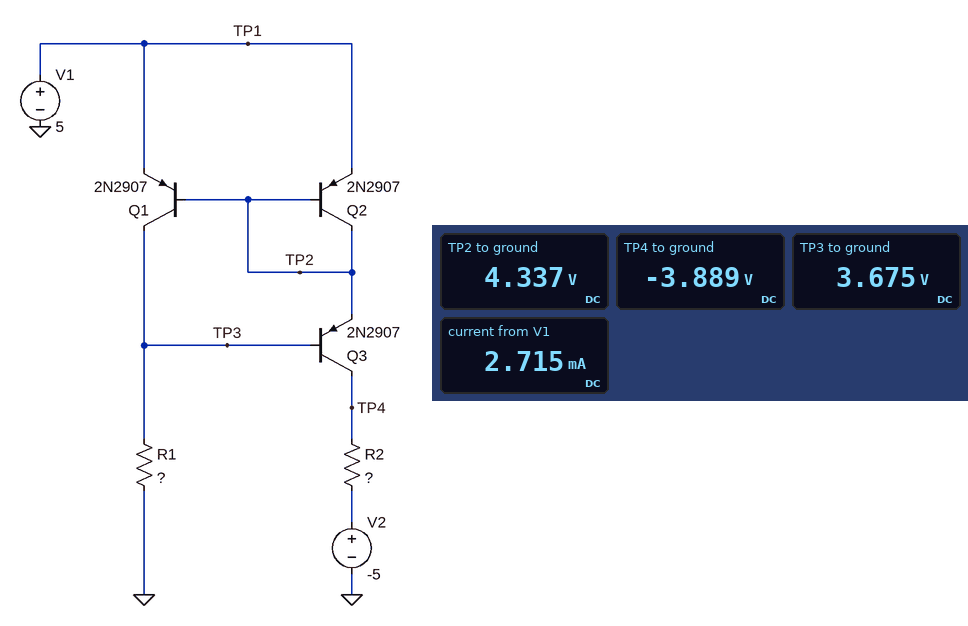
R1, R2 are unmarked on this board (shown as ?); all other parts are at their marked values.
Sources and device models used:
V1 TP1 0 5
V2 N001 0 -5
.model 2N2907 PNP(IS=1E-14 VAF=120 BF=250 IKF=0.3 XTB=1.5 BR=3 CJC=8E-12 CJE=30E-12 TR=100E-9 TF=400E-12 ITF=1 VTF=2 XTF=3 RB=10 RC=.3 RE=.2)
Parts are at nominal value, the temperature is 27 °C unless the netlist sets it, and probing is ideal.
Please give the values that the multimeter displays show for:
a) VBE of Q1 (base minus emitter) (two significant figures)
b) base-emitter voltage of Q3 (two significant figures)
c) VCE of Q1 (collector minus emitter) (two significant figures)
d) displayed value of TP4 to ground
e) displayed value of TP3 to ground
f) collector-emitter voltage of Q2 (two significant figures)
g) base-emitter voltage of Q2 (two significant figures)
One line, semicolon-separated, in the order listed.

-660 mV; -660 mV; -1.3 V; -3.889 V; 3.675 V; -660 mV; -660 mV
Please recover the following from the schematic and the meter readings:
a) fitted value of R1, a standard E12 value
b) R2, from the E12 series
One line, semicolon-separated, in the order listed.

2.7 kΩ; 820 Ω
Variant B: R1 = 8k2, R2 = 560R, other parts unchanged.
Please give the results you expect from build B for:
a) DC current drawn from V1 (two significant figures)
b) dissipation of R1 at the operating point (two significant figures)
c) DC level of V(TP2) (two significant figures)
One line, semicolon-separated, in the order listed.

910 µA; 1.7 mW; 4.4 V
